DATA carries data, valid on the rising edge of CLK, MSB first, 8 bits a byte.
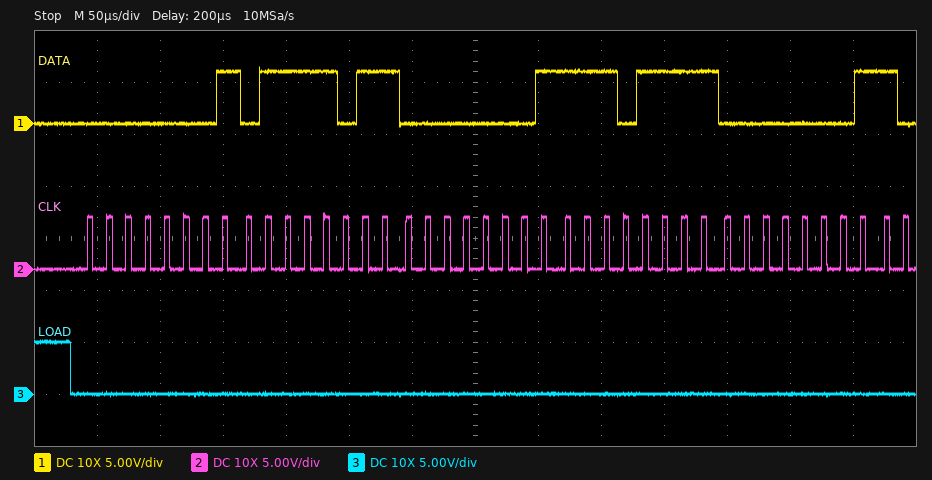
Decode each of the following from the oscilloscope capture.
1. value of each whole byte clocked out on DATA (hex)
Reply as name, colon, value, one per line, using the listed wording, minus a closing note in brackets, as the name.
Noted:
value of each whole byte clocked out on DATA: 01 7B 01 EF 01
